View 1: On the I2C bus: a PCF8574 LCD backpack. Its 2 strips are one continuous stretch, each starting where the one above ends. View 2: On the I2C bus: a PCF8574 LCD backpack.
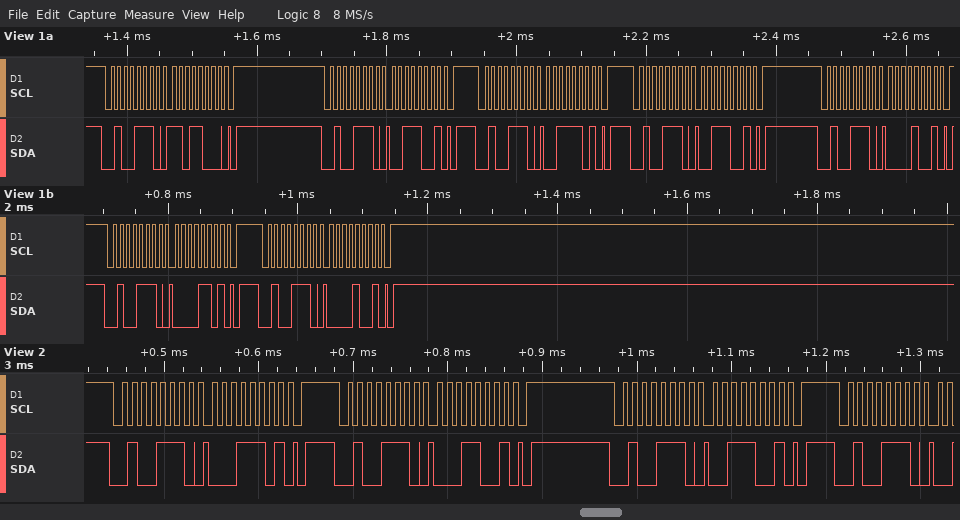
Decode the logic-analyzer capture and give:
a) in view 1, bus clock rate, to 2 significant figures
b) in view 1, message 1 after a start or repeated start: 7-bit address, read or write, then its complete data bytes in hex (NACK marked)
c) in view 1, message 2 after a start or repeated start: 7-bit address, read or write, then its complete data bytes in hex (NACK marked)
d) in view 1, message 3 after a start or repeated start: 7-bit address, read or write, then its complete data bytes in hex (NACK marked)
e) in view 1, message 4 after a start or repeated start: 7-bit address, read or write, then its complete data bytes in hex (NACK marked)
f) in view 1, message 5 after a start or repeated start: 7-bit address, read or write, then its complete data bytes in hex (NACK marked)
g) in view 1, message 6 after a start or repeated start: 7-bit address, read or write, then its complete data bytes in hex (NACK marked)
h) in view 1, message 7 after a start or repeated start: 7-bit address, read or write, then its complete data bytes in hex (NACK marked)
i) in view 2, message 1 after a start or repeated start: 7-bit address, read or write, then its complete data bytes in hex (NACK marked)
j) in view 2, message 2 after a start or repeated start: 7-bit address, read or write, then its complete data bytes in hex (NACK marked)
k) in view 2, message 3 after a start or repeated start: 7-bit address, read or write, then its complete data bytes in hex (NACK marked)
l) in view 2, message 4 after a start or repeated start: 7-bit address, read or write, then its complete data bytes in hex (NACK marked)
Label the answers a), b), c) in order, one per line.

a) 100 kHz
b) 0x27 write: D8
c) 0x27 write: 39
d) 0x27 write: 3D
e) 0x27 write: 39
f) 0x27 write: 09
g) 0x27 write: 0D
h) 0x27 write: 09
i) 0x27 write: 1D
j) 0x27 write: 19
k) 0x27 write: 39
l) 0x27 write
